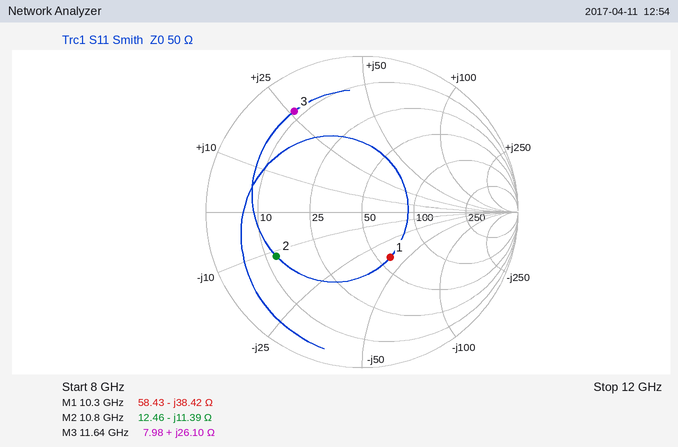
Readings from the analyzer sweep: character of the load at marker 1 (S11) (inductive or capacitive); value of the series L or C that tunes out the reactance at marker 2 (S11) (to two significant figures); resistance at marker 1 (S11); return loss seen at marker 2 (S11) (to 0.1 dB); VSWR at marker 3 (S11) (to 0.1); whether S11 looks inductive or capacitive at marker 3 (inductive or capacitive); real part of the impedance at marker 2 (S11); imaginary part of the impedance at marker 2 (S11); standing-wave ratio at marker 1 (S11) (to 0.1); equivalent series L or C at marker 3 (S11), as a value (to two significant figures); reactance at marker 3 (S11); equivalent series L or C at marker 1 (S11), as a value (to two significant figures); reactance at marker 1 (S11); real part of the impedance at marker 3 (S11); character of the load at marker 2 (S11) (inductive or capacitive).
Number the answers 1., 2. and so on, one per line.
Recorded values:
1. capacitive
2. 170 pH
3. 58.43 Ω
4. 4.2 dB
5. 8.0
6. inductive
7. 12.46 Ω
8. -11.39 Ω
9. 2.0
10. 360 pH
11. +26.10 Ω
12. 400 fF
13. -38.42 Ω
14. 7.98 Ω
15. capacitive
